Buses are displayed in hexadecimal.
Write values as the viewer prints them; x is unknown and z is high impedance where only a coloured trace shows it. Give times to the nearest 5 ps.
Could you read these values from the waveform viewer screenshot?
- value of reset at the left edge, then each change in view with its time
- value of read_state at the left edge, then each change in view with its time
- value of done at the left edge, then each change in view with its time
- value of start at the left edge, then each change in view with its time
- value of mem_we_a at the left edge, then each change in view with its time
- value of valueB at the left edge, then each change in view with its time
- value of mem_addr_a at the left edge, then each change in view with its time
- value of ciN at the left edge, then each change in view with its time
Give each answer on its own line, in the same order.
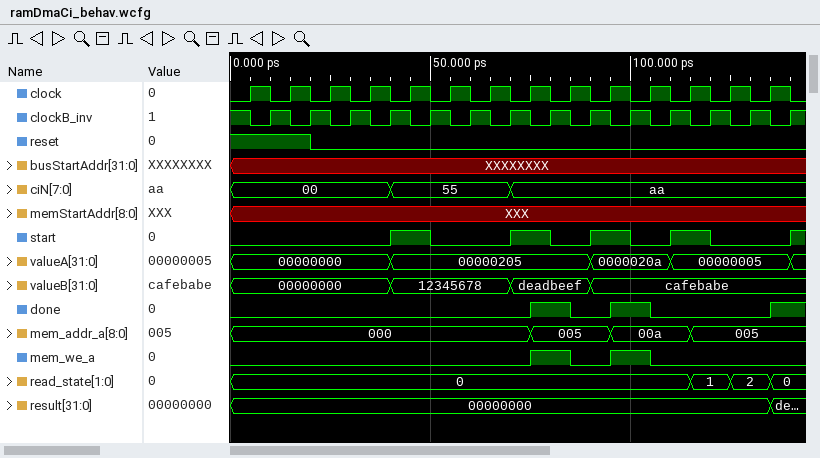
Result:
1, 0 at 20 ps
0, 1 at 115 ps, 2 at 125 ps, 0 at 135 ps
0, 1 at 75 ps, 0 at 85 ps, 1 at 95 ps, 0 at 105 ps, 1 at 135 ps
0, 1 at 40 ps, 0 at 50 ps, 1 at 70 ps, 0 at 80 ps, 1 at 90 ps, 0 at 100 ps, 1 at 110 ps, 0 at 120 ps, 1 at 140 ps
0, 1 at 75 ps, 0 at 85 ps, 1 at 95 ps, 0 at 105 ps
00000000, 12345678 at 40 ps, deadbeef at 70 ps, cafebabe at 90 ps
000, 005 at 75 ps, 00a at 95 ps, 005 at 115 ps
00, 55 at 40 ps, aa at 70 ps
